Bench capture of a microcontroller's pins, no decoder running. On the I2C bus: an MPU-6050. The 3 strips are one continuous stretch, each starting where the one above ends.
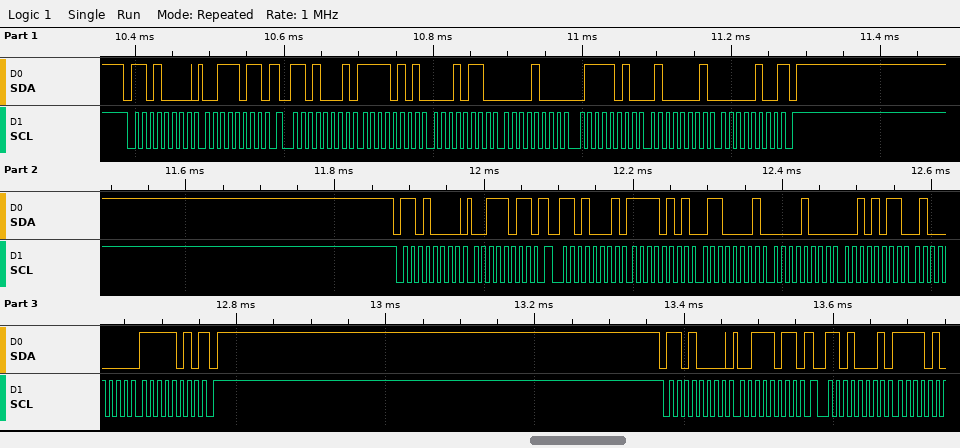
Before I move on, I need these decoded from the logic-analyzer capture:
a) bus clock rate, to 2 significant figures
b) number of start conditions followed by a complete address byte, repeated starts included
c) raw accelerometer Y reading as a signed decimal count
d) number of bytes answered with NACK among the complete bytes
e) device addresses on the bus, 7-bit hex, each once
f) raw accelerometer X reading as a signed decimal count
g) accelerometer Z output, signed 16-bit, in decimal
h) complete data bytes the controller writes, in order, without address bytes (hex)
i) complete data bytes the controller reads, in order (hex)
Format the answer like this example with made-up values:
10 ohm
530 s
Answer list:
100 kHz
6
2170
2
0x68
-2794
16644
3B 3B 3B
F5 16 08 7A 41 04 F5 61 08 2B 40 FA
